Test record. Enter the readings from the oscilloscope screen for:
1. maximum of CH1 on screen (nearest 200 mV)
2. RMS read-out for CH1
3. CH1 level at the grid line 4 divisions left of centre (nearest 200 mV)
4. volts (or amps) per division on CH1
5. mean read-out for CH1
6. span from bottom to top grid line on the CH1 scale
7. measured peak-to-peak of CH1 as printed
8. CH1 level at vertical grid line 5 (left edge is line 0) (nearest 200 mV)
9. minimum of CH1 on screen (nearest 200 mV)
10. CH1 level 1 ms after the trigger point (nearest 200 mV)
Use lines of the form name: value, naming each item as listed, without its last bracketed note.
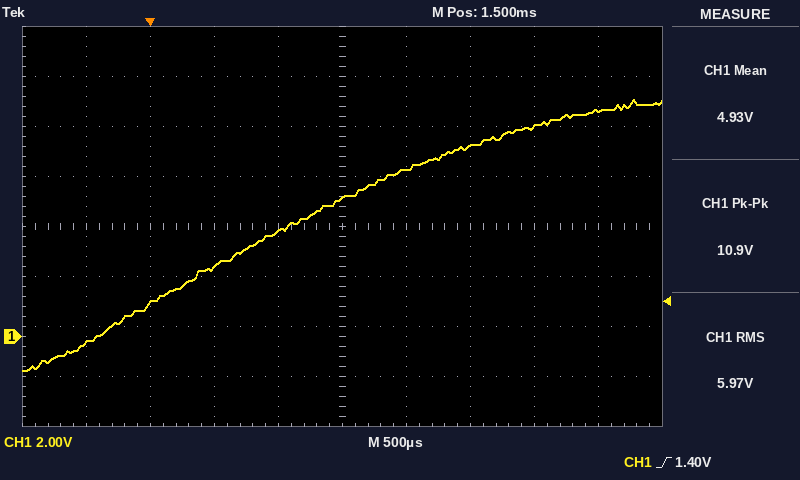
maximum of CH1 on screen: 9.4 V
RMS read-out for CH1: 5.97 V
CH1 level at the grid line 4 divisions left of centre: -200 mV
volts (or amps) per division on CH1: 2 V
mean read-out for CH1: 4.93 V
span from bottom to top grid line on the CH1 scale: 16 V
measured peak-to-peak of CH1 as printed: 10.9 V
CH1 level at vertical grid line 5 (left edge is line 0): 5.6 V
minimum of CH1 on screen: -1.4 V
CH1 level 1 ms after the trigger point: 4.2 V
